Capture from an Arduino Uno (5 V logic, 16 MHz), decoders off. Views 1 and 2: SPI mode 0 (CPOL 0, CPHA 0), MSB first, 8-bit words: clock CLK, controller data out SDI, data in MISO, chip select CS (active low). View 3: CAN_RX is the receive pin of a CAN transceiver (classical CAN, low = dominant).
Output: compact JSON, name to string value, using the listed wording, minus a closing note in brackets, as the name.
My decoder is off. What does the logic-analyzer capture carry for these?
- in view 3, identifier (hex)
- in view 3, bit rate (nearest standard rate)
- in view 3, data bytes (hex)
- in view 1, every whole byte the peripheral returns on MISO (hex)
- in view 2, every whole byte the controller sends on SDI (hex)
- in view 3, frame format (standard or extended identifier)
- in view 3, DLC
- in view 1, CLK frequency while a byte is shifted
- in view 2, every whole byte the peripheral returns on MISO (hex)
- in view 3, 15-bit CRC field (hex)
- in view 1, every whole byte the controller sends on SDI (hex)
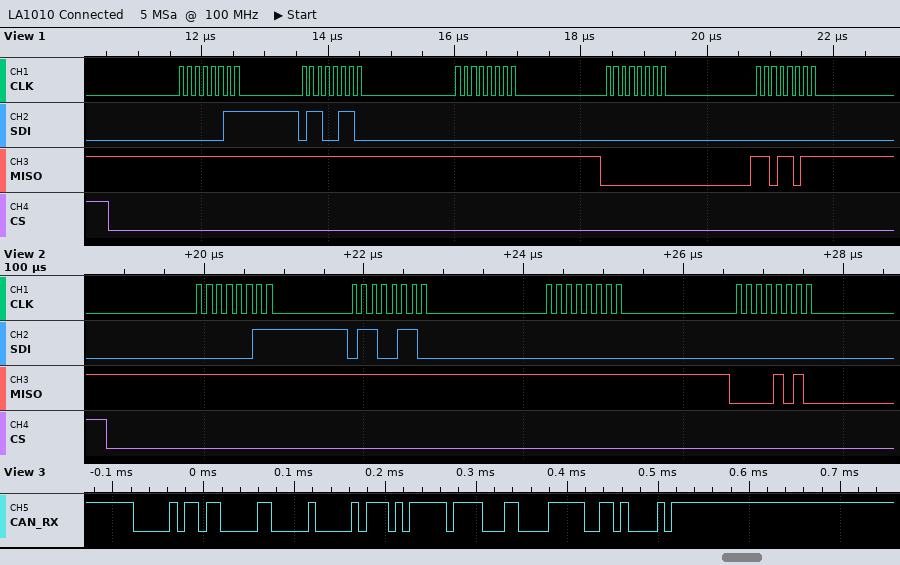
{"in view 3, identifier": "0x036", "in view 3, bit rate": "125 kbit/s", "in view 3, data bytes": "00 75 FF 18", "in view 1, every whole byte the peripheral returns on MISO": "FF FF FF 00 DB", "in view 2, every whole byte the controller sends on SDI": "03 66 00 00", "in view 3, frame format": "standard", "in view 3, DLC": "4", "in view 1, CLK frequency while a byte is shifted": "8 MHz", "in view 2, every whole byte the peripheral returns on MISO": "FF FF FF 0A", "in view 3, 15-bit CRC field": "0x3ED0", "in view 1, every whole byte the controller sends on SDI": "03 66 00 00 00"}
